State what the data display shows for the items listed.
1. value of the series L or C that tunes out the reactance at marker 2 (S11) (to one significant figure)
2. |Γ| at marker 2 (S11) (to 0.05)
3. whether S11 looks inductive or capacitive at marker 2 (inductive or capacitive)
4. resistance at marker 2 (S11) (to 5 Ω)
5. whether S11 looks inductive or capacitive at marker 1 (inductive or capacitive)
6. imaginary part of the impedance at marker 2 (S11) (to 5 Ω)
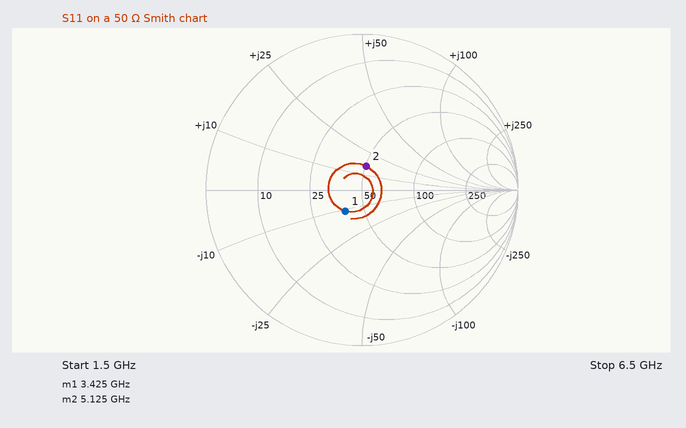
2 pF
0.15
inductive
50 Ω
capacitive
+15 Ω
